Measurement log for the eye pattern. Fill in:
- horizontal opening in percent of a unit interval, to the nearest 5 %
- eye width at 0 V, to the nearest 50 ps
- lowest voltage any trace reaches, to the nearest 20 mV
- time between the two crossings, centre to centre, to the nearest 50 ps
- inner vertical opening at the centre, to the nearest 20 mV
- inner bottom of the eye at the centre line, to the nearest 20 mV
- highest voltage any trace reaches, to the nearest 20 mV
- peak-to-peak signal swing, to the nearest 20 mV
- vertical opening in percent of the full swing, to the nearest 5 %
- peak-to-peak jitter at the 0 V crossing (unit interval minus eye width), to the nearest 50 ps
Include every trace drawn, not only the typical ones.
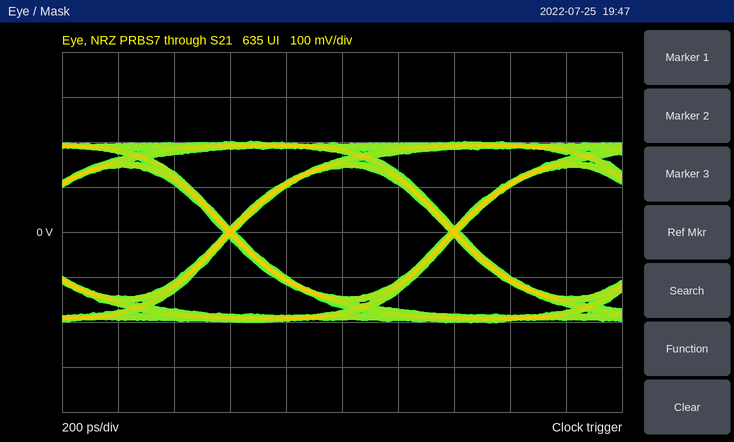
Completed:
95 %
750 ps
-200 mV
800 ps
280 mV
-140 mV
200 mV
400 mV
70 %
50 ps
